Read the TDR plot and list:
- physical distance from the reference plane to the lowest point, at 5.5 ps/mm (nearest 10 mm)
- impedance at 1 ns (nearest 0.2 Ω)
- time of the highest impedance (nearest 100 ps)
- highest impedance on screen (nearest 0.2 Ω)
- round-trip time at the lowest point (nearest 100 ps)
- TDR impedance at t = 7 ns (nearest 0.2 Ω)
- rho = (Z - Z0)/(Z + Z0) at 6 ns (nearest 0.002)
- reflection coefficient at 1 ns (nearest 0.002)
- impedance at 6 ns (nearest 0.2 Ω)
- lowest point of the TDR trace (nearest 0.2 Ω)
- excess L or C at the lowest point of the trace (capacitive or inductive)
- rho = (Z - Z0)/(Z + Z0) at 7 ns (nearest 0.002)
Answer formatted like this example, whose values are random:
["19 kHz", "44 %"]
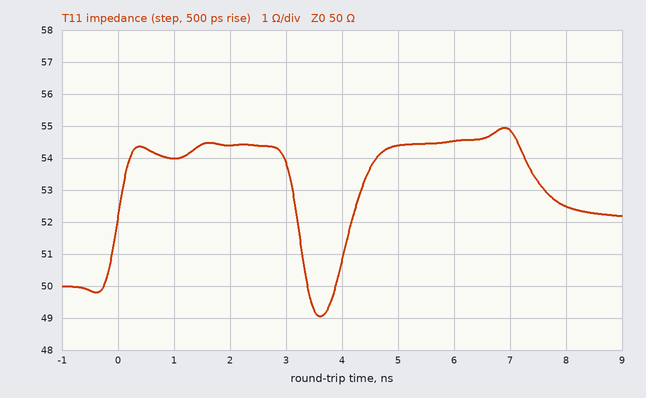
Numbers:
["330 mm", "54.0 Ω", "6.9 ns", "55.0 Ω", "3.6 ns", "54.8 Ω", "+0.044", "+0.038", "54.6 Ω", "49.0 Ω", "capacitive", "+0.046"]
